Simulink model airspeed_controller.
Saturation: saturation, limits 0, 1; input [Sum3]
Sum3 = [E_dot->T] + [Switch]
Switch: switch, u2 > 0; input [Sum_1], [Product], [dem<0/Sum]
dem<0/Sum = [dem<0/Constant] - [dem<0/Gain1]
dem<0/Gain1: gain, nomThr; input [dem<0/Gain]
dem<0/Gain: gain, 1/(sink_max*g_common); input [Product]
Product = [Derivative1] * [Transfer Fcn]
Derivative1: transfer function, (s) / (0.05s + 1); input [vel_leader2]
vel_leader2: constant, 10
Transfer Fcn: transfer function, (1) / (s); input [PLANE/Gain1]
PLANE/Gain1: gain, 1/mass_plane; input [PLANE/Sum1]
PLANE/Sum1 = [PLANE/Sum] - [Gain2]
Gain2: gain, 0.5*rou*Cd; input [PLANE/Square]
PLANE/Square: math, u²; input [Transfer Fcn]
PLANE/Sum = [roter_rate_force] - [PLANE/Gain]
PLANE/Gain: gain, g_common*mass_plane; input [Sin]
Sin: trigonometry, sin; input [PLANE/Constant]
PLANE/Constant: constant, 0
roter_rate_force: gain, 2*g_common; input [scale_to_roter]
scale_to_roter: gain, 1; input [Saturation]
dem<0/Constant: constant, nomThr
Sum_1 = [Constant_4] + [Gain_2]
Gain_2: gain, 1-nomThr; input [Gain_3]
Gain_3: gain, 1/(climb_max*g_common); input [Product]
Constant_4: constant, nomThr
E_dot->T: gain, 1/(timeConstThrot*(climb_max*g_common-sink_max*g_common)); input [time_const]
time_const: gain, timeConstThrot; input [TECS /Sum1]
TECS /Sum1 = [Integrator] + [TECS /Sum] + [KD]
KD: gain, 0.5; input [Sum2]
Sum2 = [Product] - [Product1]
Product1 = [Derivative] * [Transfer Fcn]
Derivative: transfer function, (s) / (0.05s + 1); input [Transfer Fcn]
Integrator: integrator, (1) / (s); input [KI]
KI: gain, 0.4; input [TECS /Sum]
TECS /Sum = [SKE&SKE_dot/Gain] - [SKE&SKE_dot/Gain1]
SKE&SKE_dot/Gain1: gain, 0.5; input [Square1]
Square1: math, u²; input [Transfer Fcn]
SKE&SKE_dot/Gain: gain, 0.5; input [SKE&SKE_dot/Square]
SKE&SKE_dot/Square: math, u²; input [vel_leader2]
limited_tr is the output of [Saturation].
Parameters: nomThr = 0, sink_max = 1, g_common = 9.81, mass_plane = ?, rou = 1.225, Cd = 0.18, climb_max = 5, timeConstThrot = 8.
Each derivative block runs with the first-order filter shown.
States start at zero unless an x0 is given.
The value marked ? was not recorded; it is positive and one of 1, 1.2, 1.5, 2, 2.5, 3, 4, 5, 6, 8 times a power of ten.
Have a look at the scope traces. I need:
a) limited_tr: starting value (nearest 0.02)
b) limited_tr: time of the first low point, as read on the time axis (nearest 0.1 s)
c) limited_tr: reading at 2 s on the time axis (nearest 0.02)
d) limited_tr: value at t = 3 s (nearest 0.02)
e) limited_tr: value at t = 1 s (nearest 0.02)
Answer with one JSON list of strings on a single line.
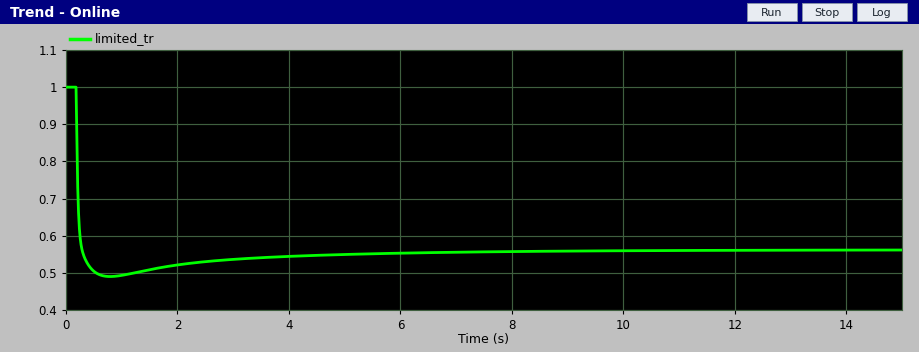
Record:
["1.00", "0.8 s", "0.52", "0.54", "0.50"]
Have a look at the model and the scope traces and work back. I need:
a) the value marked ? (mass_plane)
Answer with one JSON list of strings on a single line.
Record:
["1"]
